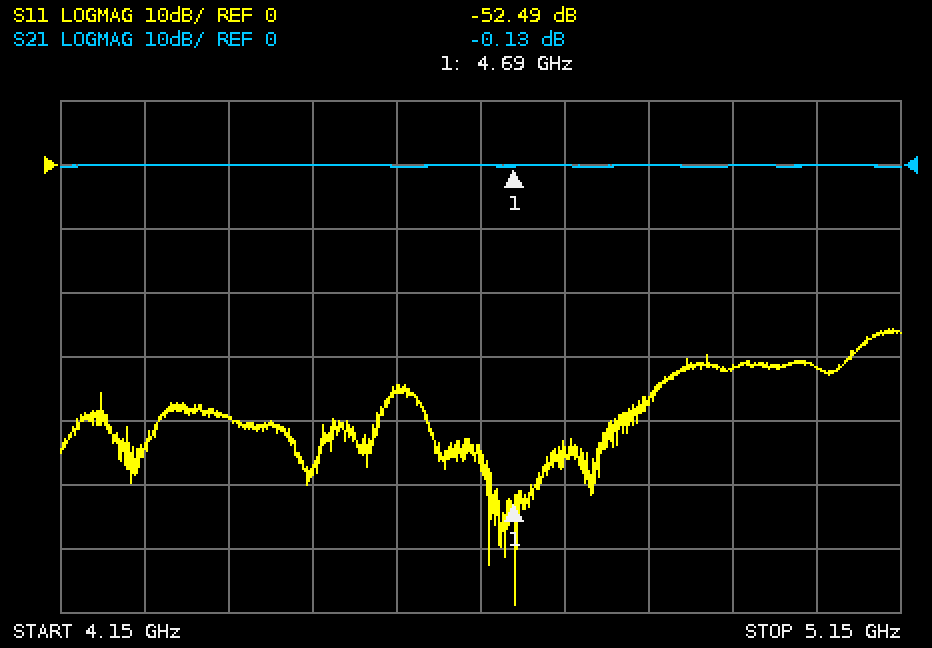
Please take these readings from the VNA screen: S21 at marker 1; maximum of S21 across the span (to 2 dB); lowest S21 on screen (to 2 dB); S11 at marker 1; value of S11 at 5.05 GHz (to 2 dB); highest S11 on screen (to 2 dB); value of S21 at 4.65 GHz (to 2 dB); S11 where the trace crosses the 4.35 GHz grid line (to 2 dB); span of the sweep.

-0.13 dB
0 dB
0 dB
-52.49 dB
-32 dB
-26 dB
0 dB
-40 dB
1 GHz
